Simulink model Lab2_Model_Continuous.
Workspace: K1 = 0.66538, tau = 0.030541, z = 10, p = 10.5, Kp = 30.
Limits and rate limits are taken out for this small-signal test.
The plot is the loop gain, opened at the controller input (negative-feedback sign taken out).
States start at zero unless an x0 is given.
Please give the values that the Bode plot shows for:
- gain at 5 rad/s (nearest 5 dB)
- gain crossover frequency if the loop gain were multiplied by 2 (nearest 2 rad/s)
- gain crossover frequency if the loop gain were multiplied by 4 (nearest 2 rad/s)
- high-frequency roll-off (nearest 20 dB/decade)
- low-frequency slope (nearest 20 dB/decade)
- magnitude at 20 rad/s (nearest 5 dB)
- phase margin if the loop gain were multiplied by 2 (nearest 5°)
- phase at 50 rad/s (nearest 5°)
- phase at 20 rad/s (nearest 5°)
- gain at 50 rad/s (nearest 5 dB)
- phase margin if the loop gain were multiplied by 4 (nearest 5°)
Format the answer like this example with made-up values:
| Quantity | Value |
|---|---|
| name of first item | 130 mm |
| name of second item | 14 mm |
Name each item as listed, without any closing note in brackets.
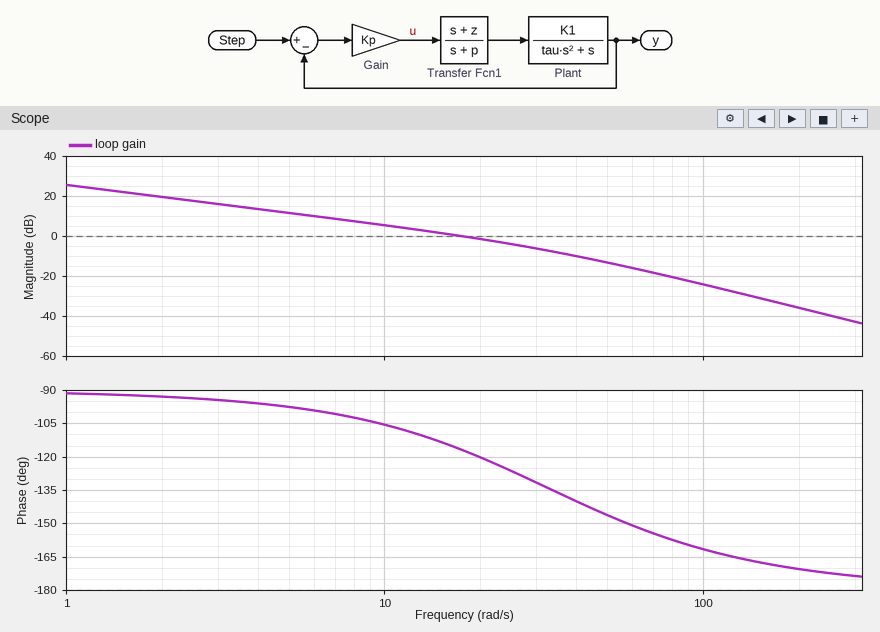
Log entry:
| Quantity | Value |
|---|---|
| gain at 5 rad/s | 10 dB |
| gain crossover frequency if the loop gain were multiplied by 2 | 30 rad/s |
| gain crossover frequency if the loop gain were multiplied by 4 | 46 rad/s |
| high-frequency roll-off | -40 dB/decade |
| low-frequency slope | -20 dB/decade |
| magnitude at 20 rad/s | 0 dB |
| phase margin if the loop gain were multiplied by 2 | 50° |
| phase at 50 rad/s | -145° |
| phase at 20 rad/s | -120° |
| gain at 50 rad/s | -15 dB |
| phase margin if the loop gain were multiplied by 4 | 35° |
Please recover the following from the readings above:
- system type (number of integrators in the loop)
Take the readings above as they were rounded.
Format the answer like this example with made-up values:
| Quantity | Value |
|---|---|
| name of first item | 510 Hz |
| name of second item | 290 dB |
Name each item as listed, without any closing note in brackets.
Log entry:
| Quantity | Value |
|---|---|
| system type | 1 |
